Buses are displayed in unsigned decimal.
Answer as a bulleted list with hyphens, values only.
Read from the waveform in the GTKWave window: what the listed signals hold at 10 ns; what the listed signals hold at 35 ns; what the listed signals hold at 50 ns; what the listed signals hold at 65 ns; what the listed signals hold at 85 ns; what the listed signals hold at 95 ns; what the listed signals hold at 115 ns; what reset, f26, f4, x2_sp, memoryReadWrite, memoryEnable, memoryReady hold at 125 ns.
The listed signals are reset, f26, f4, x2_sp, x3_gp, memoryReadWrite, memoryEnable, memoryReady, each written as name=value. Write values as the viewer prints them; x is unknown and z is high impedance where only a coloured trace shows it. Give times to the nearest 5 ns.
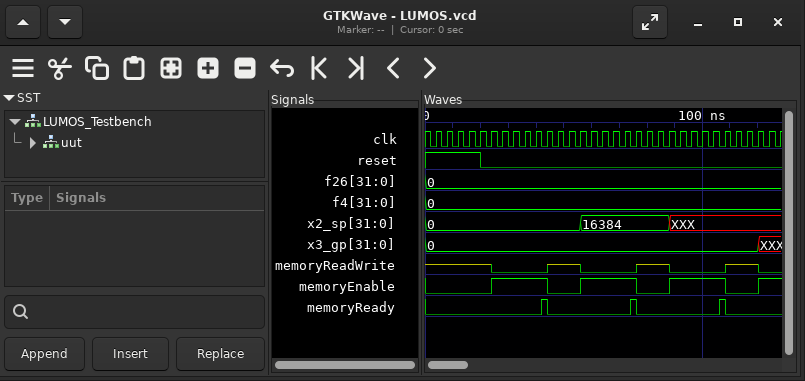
- reset=1, f26=0, f4=0, x2_sp=0, x3_gp=0, memoryReadWrite=z, memoryEnable=0, memoryReady=0
- reset=0, f26=0, f4=0, x2_sp=0, x3_gp=0, memoryReadWrite=0, memoryEnable=1, memoryReady=0
- reset=0, f26=0, f4=0, x2_sp=0, x3_gp=0, memoryReadWrite=z, memoryEnable=0, memoryReady=0
- reset=0, f26=0, f4=0, x2_sp=16384, x3_gp=0, memoryReadWrite=0, memoryEnable=1, memoryReady=0
- reset=0, f26=0, f4=0, x2_sp=16384, x3_gp=0, memoryReadWrite=z, memoryEnable=0, memoryReady=0
- reset=0, f26=0, f4=0, x2_sp=XXX, x3_gp=0, memoryReadWrite=0, memoryEnable=1, memoryReady=0
- reset=0, f26=0, f4=0, x2_sp=XXX, x3_gp=0, memoryReadWrite=z, memoryEnable=0, memoryReady=0
- reset=0, f26=0, f4=0, x2_sp=XXX, memoryReadWrite=0, memoryEnable=1, memoryReady=0
